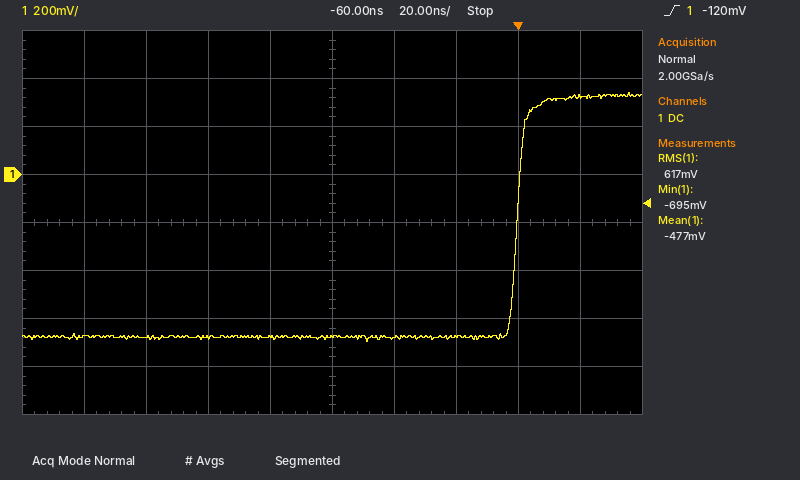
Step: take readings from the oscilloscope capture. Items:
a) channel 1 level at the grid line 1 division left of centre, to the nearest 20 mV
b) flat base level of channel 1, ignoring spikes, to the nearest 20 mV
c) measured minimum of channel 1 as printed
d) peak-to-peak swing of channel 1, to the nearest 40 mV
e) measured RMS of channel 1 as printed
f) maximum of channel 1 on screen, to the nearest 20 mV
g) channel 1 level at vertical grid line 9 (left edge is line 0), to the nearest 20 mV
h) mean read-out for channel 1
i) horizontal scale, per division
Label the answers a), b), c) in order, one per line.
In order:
a) -680 mV
b) -680 mV
c) -695 mV
d) 1.04 V
e) 617 mV
f) 340 mV
g) 320 mV
h) -477 mV
i) 20 ns
